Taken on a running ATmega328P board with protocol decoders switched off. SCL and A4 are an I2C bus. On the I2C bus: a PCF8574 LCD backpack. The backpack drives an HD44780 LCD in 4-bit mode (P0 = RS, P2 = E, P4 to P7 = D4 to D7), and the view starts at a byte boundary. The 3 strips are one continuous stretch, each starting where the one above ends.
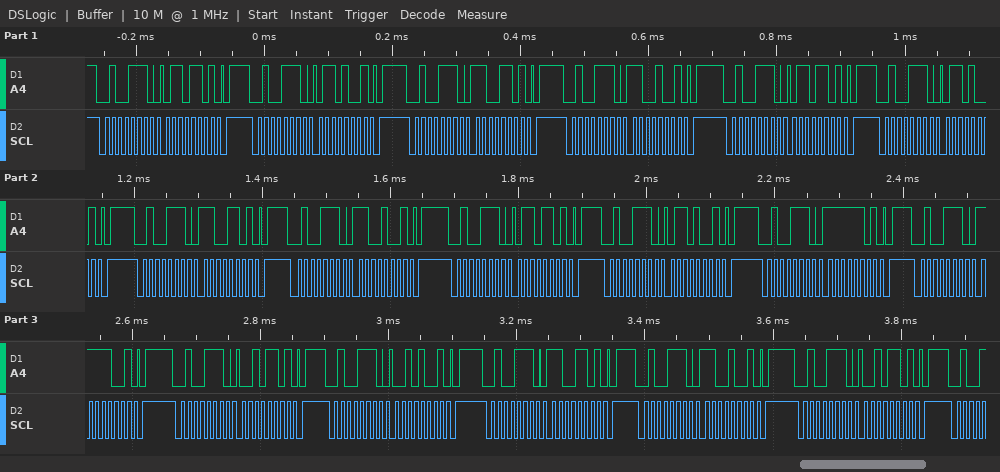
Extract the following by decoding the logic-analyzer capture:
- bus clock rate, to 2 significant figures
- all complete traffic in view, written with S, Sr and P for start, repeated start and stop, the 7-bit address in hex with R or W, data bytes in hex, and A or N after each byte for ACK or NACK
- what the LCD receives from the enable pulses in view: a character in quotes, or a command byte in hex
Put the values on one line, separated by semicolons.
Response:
100 kHz; S 27W A 6D A P S 27W A 69 A P S 27W A CD A P S 27W A C9 A P S 27W A 6D A P S 27W A 69 A P S 27W A CD A P S 27W A C9 A P S 27W A 6D A P S 27W A 69 A P S 27W A FD A P S 27W A F9 A P S 27W A 2D A P S 27W A 29 A P S 27W A CD A P S 27W A C9 A P S 27W A 2D A P; 'l' 'l' 'o' ','
